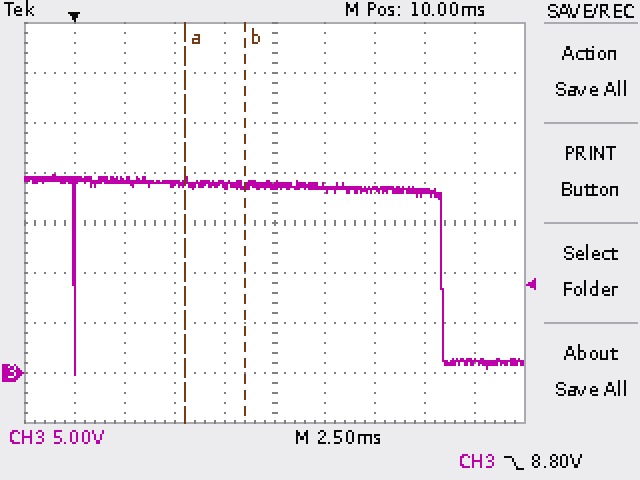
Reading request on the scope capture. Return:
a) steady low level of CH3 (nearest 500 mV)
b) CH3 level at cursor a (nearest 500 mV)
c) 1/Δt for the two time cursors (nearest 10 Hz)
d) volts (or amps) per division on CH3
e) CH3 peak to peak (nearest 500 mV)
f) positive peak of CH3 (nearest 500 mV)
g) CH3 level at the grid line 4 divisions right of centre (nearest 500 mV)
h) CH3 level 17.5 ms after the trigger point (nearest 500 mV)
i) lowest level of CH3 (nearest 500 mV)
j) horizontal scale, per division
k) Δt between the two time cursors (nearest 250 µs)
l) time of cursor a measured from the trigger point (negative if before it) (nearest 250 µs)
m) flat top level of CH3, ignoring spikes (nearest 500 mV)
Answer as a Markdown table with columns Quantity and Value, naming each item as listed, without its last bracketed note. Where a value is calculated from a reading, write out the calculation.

| Quantity | Value |
|---|---|
| steady low level of CH3 | 1.0 V |
| CH3 level at cursor a | 19.0 V |
| 1/Δt for the two time cursors | 1 / 3.00 ms ≈ 330 Hz |
| volts (or amps) per division on CH3 | 5 V |
| CH3 peak to peak | 20.0 V − (0.0 V) = 20.0 V |
| positive peak of CH3 | 20.0 V |
| CH3 level at the grid line 4 divisions right of centre | 1.0 V |
| CH3 level 17.5 ms after the trigger point | 18.0 V |
| lowest level of CH3 | 0.0 V |
| horizontal scale, per division | 2.5 ms |
| Δt between the two time cursors | 3.00 ms |
| time of cursor a measured from the trigger point (negative if before it) | +5.50 ms |
| flat top level of CH3, ignoring spikes | 19.0 V |
